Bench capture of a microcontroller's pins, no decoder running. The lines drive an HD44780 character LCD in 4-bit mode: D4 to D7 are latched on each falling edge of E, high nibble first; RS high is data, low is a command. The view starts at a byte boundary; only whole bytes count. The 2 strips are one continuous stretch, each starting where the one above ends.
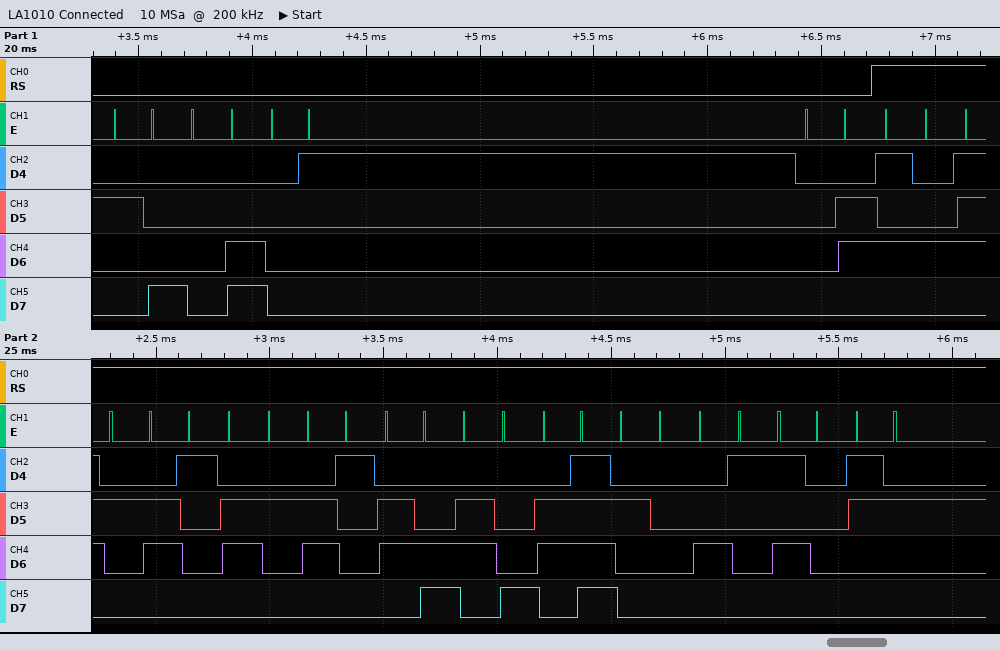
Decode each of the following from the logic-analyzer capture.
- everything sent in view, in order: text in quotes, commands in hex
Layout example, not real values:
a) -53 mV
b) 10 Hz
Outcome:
a) 0x28 0x0C 0x01 0x06 "Trabalho AP2"
